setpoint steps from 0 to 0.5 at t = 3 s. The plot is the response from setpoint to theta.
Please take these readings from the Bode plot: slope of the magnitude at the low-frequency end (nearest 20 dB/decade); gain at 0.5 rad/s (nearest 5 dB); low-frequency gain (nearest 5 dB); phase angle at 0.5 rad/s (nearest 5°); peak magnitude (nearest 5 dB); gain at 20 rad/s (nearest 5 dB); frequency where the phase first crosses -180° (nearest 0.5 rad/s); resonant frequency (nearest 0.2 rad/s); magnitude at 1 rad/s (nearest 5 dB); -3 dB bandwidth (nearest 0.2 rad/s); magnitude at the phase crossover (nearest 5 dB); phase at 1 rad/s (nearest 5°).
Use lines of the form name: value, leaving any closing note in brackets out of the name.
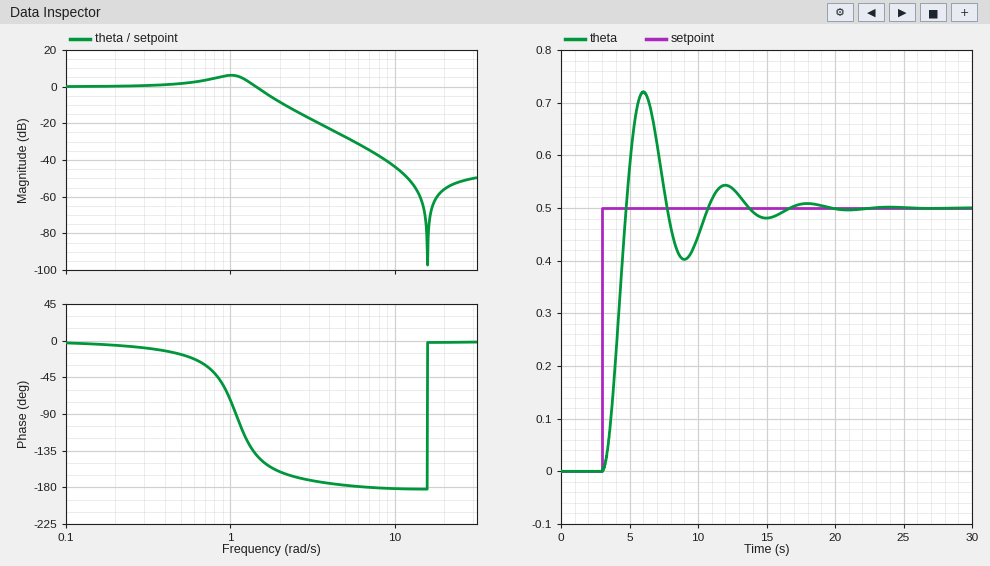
slope of the magnitude at the low-frequency end: 0 dB/decade
gain at 0.5 rad/s: 0 dB
low-frequency gain: 0 dB
phase angle at 0.5 rad/s: -15°
peak magnitude: 5 dB
gain at 20 rad/s: -55 dB
frequency where the phase first crosses -180°: 7.0 rad/s
resonant frequency: 1.0 rad/s
magnitude at 1 rad/s: 5 dB
-3 dB bandwidth: 1.6 rad/s
magnitude at the phase crossover: -35 dB
phase at 1 rad/s: -75°
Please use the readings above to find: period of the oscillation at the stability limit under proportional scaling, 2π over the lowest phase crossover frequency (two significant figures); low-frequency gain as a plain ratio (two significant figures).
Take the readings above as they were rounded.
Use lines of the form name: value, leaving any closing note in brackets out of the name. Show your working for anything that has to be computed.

period of the oscillation at the stability limit under proportional scaling, 2π over the lowest phase crossover frequency: 2π / 7 = 0.90 s
low-frequency gain as a plain ratio: 10^(0 / 20) = 1.0
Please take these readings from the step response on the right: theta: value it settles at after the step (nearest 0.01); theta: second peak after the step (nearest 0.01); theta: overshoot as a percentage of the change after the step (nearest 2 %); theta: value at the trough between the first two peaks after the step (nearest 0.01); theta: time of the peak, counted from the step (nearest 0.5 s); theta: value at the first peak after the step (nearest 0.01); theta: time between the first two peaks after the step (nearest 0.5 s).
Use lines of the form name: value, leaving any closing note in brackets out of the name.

theta: value it settles at after the step: 0.50
theta: second peak after the step: 0.54
theta: overshoot as a percentage of the change after the step: 44 %
theta: value at the trough between the first two peaks after the step: 0.40
theta: time of the peak, counted from the step: 3.0 s
theta: value at the first peak after the step: 0.72
theta: time between the first two peaks after the step: 6.0 s
